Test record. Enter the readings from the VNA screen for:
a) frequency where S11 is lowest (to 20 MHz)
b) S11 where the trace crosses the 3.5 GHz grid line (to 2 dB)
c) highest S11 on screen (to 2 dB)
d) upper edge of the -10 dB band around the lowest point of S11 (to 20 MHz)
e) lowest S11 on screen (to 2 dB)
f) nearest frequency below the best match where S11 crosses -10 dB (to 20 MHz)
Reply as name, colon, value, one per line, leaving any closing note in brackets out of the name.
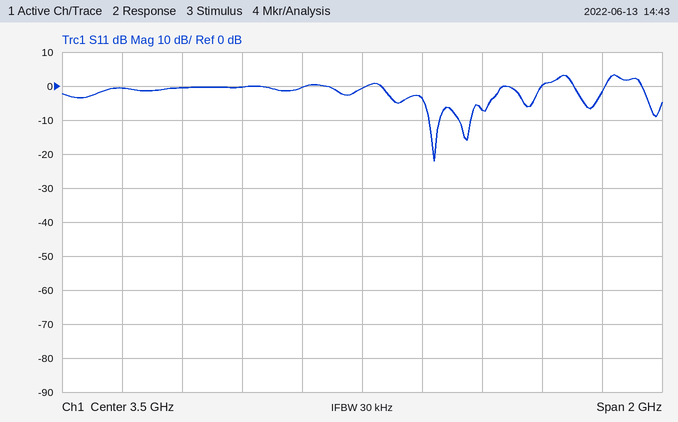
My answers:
frequency where S11 is lowest: 3.74 GHz
S11 where the trace crosses the 3.5 GHz grid line: 0 dB
highest S11 on screen: 4 dB
upper edge of the -10 dB band around the lowest point of S11: 3.76 GHz
lowest S11 on screen: -22 dB
nearest frequency below the best match where S11 crosses -10 dB: 3.72 GHz
